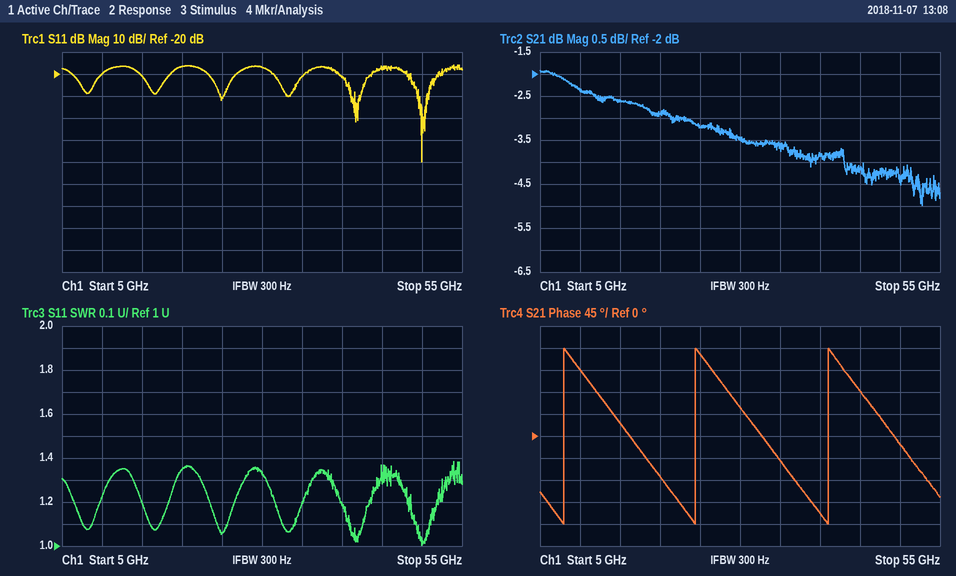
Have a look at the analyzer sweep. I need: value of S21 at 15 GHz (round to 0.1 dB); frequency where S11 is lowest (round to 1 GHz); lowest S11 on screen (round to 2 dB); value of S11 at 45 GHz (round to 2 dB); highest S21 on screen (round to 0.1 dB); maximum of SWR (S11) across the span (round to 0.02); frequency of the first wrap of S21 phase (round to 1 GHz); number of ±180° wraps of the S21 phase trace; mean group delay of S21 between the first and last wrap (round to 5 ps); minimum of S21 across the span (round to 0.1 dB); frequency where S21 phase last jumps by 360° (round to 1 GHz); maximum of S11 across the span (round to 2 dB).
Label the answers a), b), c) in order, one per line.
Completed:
a) -2.6 dB
b) 50 GHz
c) -60 dB
d) -18 dB
e) -1.9 dB
f) 1.38
g) 8 GHz
h) 3
i) 60 ps
j) -5.0 dB
k) 41 GHz
l) -16 dB
